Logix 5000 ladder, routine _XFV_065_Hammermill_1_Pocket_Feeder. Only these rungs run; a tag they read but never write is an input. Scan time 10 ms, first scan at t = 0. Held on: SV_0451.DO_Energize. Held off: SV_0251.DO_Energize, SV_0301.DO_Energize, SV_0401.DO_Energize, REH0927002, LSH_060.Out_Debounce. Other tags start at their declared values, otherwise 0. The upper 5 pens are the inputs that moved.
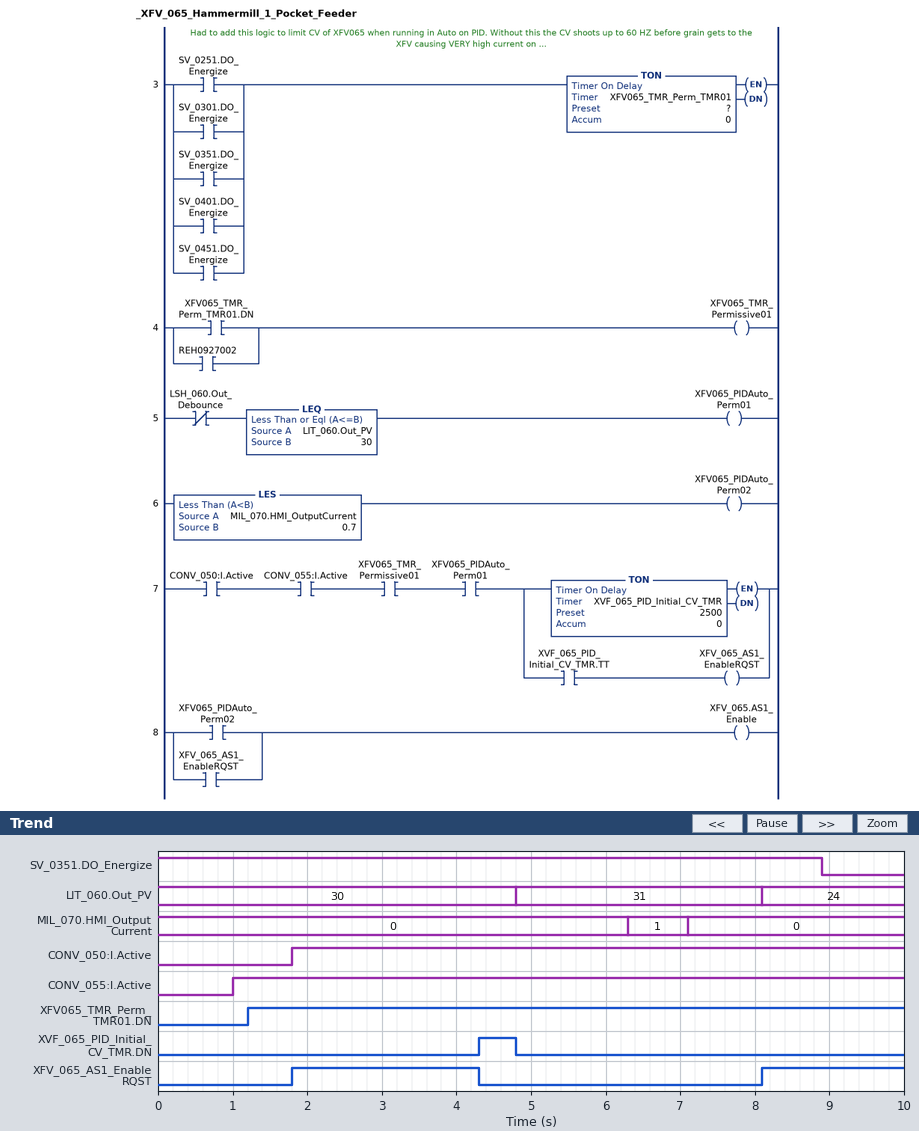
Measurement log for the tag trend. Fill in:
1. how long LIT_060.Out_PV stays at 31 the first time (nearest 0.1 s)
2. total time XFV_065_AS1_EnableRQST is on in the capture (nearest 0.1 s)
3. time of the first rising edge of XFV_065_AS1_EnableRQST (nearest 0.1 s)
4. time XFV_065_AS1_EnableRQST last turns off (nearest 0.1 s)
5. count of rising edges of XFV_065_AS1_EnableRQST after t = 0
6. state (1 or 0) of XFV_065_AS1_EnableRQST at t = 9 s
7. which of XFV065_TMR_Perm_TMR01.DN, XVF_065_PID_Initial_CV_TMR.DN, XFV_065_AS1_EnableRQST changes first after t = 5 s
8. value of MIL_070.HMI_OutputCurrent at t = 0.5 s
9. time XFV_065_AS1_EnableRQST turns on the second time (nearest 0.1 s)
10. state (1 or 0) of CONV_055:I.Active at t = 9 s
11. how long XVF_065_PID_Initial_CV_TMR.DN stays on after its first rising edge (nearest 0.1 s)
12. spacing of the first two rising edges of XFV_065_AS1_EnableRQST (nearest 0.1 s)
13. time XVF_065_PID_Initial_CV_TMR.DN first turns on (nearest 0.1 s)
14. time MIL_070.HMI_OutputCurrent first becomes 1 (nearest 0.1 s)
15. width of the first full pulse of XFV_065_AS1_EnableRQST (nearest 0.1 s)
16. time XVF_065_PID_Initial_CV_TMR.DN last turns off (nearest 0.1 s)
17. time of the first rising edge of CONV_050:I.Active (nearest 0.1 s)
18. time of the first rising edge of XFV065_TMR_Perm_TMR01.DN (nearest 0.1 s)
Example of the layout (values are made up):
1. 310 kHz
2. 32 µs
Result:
1. 3.3 s
2. 4.4 s
3. 1.8 s
4. 4.3 s
5. 2
6. 1
7. XFV_065_AS1_EnableRQST
8. 0
9. 8.1 s
10. 1
11. 0.5 s
12. 6.3 s
13. 4.3 s
14. 6.3 s
15. 2.5 s
16. 4.8 s
17. 1.8 s
18. 1.2 s
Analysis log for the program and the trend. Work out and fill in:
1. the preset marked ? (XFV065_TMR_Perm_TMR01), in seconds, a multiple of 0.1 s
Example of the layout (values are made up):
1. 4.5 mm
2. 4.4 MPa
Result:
1. 1.2 s
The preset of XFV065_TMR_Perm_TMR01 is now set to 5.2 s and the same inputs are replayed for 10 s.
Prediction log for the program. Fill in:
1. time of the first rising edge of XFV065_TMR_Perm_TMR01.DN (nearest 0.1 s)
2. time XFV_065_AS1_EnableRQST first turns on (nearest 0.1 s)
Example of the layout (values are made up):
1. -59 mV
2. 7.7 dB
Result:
1. 5.2 s
2. 8.1 s
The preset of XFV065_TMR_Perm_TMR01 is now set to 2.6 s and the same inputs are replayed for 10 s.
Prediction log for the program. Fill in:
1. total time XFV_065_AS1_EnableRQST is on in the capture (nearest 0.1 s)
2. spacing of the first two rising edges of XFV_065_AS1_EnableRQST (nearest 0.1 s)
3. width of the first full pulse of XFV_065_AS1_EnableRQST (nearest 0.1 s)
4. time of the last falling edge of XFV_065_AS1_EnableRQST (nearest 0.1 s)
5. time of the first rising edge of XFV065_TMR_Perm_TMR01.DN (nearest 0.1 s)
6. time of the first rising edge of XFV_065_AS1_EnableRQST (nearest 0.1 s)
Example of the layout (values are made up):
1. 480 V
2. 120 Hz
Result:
1. 4.1 s
2. 5.5 s
3. 2.2 s
4. 4.8 s
5. 2.6 s
6. 2.6 s
